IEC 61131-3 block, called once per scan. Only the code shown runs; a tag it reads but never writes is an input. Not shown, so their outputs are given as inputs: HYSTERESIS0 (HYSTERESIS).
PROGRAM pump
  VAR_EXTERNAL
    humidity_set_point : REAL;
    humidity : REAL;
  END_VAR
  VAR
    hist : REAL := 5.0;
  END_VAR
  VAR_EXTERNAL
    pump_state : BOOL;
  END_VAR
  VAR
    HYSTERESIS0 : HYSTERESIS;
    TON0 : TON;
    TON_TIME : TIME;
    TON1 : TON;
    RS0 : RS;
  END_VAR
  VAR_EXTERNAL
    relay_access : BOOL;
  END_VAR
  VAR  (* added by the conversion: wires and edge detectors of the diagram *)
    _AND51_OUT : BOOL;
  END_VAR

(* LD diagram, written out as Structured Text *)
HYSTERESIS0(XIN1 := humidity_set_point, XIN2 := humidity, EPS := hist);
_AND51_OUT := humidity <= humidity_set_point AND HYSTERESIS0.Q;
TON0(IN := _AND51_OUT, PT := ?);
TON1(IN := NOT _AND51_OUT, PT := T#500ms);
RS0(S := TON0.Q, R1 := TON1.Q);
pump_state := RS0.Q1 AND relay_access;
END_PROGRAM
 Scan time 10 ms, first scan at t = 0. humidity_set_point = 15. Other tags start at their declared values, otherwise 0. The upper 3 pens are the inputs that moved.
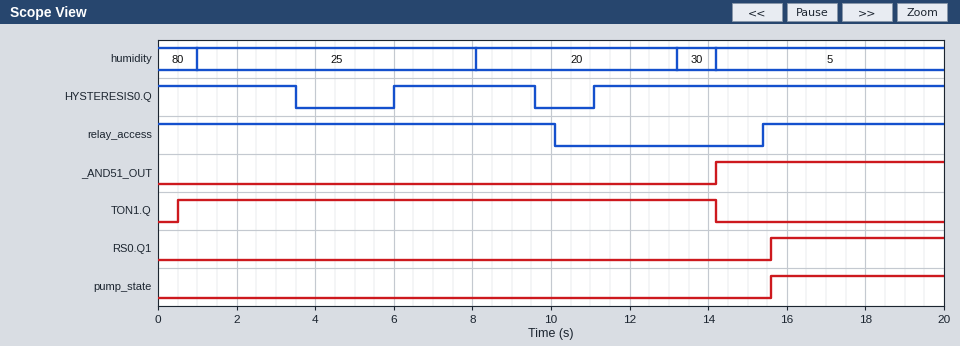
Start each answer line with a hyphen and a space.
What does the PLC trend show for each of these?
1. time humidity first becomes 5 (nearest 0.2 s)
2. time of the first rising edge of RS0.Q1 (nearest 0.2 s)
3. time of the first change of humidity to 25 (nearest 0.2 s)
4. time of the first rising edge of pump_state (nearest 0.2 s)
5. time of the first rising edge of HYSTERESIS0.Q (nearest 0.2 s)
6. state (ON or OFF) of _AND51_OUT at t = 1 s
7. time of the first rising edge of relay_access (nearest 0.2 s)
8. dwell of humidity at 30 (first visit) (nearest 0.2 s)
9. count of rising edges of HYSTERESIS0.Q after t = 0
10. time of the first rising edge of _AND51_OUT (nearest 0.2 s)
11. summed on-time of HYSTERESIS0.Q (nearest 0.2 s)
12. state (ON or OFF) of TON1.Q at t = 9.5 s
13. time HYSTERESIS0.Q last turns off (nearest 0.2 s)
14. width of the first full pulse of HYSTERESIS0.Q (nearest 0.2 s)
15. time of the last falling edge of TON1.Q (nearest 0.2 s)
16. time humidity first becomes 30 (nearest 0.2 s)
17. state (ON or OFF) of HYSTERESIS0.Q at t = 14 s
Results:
- 14.2 s
- 15.6 s
- 1.0 s
- 15.6 s
- 6.0 s
- OFF
- 15.4 s
- 1.0 s
- 2
- 14.2 s
- 16.0 s
- ON
- 9.6 s
- 3.6 s
- 14.2 s
- 13.2 s
- ON
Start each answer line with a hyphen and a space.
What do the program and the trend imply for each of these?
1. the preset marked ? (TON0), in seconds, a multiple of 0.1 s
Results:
- 1.4 s
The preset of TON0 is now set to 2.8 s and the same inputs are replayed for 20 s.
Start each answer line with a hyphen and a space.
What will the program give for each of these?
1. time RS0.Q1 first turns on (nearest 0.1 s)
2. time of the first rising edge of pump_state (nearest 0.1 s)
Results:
- 17.0 s
- 17.0 s
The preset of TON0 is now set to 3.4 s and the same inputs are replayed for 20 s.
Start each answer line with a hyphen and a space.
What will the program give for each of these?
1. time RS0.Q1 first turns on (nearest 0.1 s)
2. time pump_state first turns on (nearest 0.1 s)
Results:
- 17.6 s
- 17.6 s
